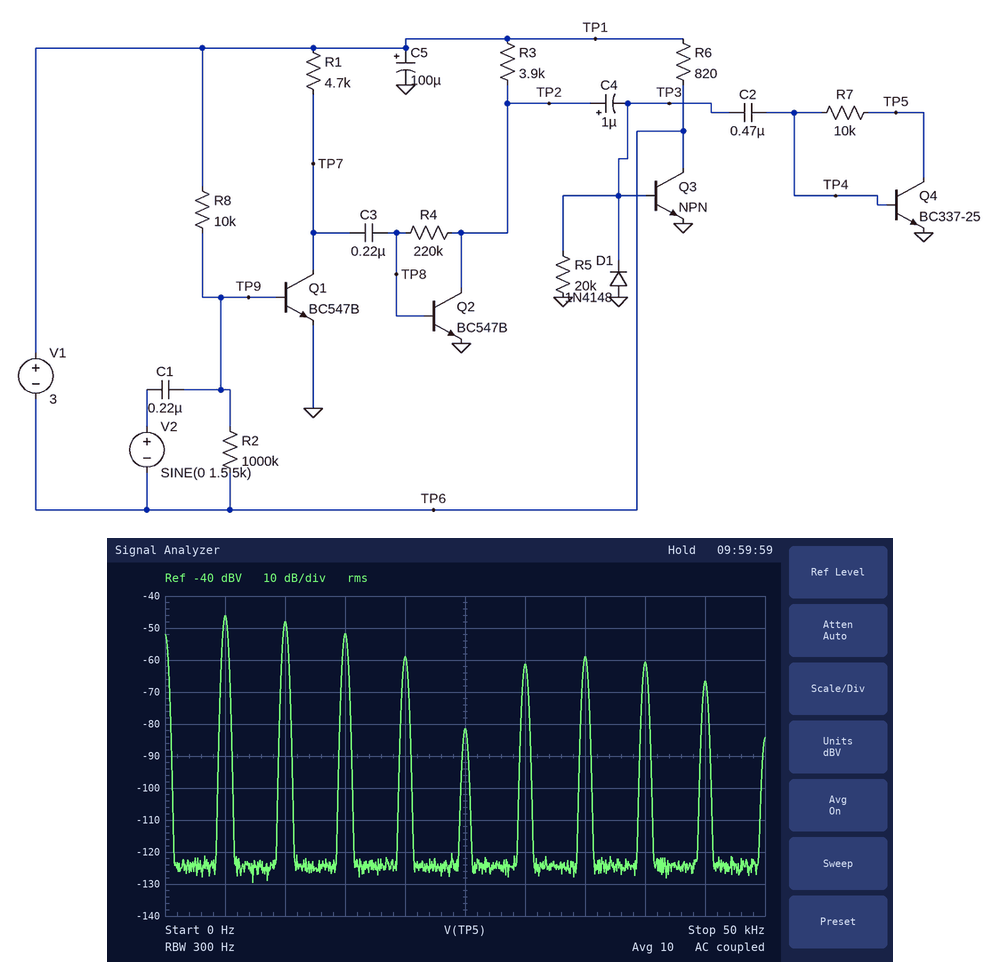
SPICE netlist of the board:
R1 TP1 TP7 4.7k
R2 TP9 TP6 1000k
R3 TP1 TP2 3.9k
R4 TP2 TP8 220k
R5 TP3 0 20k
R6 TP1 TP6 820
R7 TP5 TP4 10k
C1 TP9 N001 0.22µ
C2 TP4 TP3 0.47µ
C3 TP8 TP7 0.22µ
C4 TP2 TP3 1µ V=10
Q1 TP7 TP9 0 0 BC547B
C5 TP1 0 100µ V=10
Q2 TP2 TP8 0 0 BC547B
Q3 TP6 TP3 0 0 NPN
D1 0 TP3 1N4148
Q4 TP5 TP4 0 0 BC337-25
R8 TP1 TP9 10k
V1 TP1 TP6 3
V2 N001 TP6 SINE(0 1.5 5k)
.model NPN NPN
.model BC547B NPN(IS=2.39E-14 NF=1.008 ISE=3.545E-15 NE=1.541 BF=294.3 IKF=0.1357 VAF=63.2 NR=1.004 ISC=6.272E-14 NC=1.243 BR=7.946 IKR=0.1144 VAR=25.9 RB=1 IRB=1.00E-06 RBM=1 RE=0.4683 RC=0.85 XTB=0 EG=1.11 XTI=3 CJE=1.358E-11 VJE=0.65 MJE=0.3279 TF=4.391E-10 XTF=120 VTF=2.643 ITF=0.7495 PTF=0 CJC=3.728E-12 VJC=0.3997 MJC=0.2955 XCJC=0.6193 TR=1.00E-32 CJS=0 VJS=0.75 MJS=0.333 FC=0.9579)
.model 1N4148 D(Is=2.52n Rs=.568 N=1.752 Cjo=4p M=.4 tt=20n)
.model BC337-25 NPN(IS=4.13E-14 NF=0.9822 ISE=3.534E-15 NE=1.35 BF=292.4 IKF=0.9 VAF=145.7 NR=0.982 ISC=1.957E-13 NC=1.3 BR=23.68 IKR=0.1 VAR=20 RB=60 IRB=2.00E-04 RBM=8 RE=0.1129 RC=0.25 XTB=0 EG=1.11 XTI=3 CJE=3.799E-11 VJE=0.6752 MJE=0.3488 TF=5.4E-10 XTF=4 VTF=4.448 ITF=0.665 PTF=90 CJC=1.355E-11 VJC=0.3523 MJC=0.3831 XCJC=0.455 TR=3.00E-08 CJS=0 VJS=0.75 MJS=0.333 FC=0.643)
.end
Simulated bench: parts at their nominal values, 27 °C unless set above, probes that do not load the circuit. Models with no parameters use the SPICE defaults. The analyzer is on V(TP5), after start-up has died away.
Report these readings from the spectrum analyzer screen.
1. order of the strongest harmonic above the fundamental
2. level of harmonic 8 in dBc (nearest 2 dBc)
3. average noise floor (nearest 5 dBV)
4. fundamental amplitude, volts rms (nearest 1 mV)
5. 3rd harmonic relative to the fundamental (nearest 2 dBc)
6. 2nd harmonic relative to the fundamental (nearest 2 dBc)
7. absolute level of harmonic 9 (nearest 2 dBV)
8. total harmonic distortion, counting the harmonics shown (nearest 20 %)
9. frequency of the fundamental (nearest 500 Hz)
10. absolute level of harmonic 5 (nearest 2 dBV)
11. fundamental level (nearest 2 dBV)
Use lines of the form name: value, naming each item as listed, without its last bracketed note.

order of the strongest harmonic above the fundamental: 2
level of harmonic 8 in dBc: -14 dBc
average noise floor: -125 dBV
fundamental amplitude, volts rms: 5 mV
3rd harmonic relative to the fundamental: -6 dBc
2nd harmonic relative to the fundamental: -2 dBc
absolute level of harmonic 9: -66 dBV
total harmonic distortion, counting the harmonics shown: 100 %
frequency of the fundamental: 5.0 kHz
absolute level of harmonic 5: -82 dBV
fundamental level: -46 dBV
